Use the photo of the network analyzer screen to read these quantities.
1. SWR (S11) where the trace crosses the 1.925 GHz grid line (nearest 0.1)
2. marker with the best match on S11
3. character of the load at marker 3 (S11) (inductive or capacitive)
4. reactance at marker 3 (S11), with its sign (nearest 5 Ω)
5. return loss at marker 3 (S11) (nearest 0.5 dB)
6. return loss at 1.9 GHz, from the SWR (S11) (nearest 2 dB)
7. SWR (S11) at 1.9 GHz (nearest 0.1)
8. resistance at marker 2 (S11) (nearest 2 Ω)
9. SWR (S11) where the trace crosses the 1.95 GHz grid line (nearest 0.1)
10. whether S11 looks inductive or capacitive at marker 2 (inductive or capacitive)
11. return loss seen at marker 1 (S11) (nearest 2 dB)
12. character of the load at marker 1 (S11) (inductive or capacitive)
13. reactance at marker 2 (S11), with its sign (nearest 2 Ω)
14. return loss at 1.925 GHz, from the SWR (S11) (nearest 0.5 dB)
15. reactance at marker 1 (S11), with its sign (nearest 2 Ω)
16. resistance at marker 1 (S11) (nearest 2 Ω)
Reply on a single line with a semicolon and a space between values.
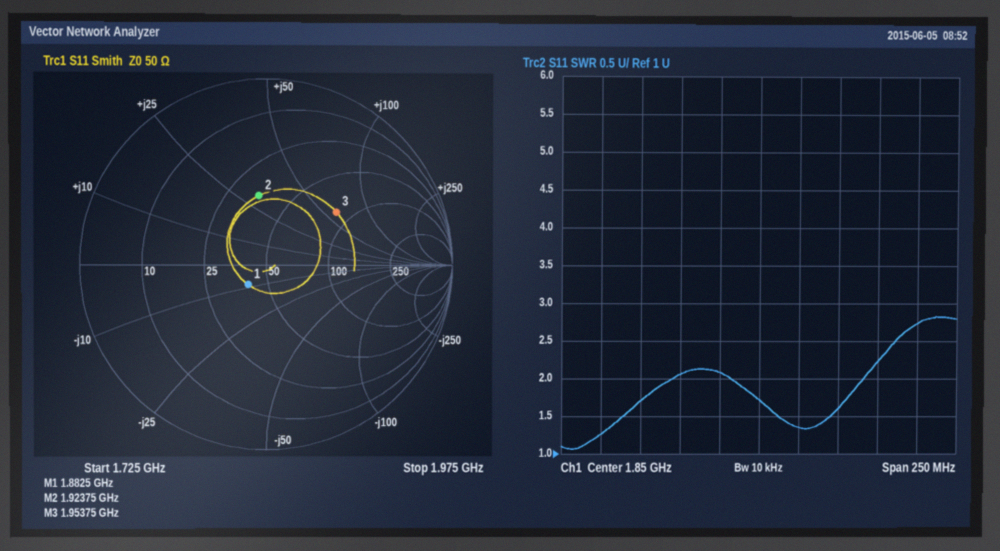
2.2; marker 1; inductive; +60 Ω; 6.5 dB; 12 dB; 1.6; 36 Ω; 2.7; inductive; 16 dB; capacitive; +30 Ω; 8.5 dB; -8 Ω; 40 Ω
